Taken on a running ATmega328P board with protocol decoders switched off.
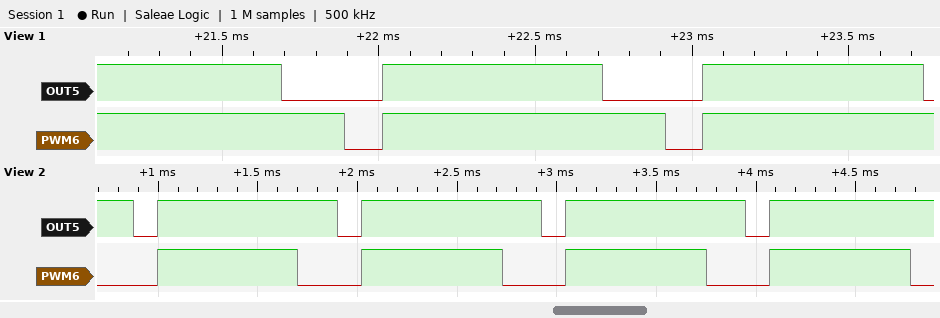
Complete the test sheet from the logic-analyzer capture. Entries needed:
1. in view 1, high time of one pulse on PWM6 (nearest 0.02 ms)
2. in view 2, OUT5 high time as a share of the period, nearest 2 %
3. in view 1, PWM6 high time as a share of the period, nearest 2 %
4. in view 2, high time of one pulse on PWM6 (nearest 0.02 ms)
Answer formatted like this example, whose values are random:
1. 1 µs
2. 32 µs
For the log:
1. 0.90 ms
2. 88 %
3. 88 %
4. 0.70 ms
